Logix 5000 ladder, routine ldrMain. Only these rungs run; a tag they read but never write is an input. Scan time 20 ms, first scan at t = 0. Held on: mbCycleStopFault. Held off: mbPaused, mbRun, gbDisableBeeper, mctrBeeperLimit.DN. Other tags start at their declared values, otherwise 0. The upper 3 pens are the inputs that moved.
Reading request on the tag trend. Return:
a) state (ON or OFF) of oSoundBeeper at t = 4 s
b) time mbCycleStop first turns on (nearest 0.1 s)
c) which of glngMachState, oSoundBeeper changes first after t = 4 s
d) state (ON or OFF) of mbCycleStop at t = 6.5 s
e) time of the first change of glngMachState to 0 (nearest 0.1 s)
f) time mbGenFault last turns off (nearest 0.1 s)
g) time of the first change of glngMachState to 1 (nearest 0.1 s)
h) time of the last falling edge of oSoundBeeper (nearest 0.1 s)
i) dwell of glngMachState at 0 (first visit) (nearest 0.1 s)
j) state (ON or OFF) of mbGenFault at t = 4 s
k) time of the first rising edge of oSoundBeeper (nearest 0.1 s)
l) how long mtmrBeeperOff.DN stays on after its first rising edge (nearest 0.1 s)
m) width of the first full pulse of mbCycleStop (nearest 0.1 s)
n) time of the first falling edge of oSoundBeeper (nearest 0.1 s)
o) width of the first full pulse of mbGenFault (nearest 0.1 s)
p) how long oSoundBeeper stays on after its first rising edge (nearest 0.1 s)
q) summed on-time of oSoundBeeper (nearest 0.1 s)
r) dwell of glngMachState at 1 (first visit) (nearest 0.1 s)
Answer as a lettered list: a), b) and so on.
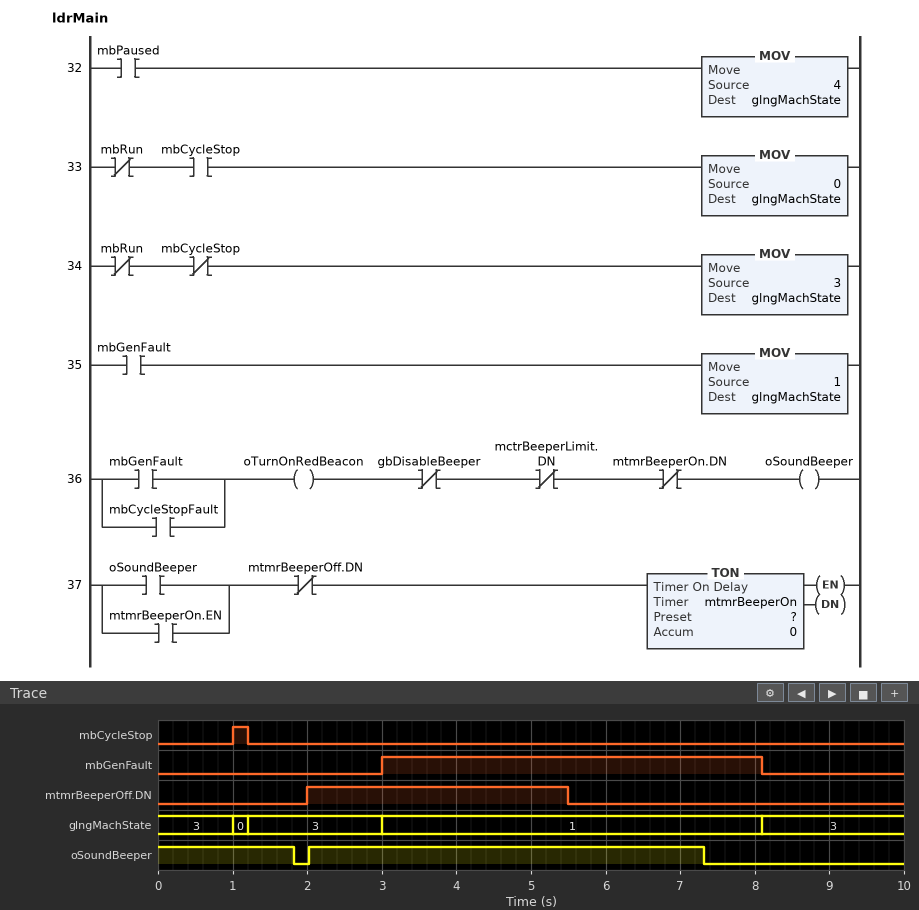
a) ON
b) 1.0 s
c) oSoundBeeper
d) OFF
e) 1.0 s
f) 8.1 s
g) 3.0 s
h) 7.3 s
i) 0.2 s
j) ON
k) 2.0 s
l) 3.5 s
m) 0.2 s
n) 1.8 s
o) 5.1 s
p) 5.3 s
q) 7.1 s
r) 5.1 s
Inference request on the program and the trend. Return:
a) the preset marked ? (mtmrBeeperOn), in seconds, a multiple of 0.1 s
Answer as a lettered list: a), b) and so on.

a) 1.8 s
